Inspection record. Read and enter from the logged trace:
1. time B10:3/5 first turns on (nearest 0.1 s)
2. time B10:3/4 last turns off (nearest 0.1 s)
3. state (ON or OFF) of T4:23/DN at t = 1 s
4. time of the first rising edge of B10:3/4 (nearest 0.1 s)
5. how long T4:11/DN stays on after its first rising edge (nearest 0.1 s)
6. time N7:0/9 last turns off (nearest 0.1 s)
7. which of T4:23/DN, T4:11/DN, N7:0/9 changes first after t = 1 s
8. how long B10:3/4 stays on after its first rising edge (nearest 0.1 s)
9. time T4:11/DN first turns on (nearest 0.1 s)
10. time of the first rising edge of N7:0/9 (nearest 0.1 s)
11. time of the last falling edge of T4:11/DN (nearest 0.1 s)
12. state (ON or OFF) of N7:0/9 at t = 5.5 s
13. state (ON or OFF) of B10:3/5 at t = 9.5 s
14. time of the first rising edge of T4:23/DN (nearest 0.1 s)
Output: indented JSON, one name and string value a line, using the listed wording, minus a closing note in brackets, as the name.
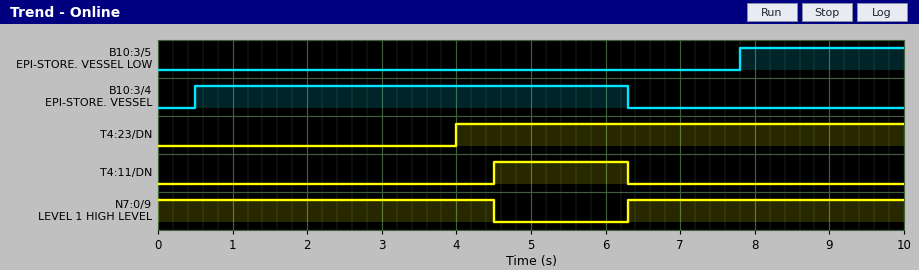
{
  "time B10:3/5 first turns on": "7.8 s",
  "time B10:3/4 last turns off": "6.3 s",
  "state (ON or OFF) of T4:23/DN at t = 1 s": "OFF",
  "time of the first rising edge of B10:3/4": "0.5 s",
  "how long T4:11/DN stays on after its first rising edge": "1.8 s",
  "time N7:0/9 last turns off": "4.5 s",
  "which of T4:23/DN, T4:11/DN, N7:0/9 changes first after t = 1 s": "T4:23/DN",
  "how long B10:3/4 stays on after its first rising edge": "5.8 s",
  "time T4:11/DN first turns on": "4.5 s",
  "time of the first rising edge of N7:0/9": "6.3 s",
  "time of the last falling edge of T4:11/DN": "6.3 s",
  "state (ON or OFF) of N7:0/9 at t = 5.5 s": "OFF",
  "state (ON or OFF) of B10:3/5 at t = 9.5 s": "ON",
  "time of the first rising edge of T4:23/DN": "4.0 s"
}
